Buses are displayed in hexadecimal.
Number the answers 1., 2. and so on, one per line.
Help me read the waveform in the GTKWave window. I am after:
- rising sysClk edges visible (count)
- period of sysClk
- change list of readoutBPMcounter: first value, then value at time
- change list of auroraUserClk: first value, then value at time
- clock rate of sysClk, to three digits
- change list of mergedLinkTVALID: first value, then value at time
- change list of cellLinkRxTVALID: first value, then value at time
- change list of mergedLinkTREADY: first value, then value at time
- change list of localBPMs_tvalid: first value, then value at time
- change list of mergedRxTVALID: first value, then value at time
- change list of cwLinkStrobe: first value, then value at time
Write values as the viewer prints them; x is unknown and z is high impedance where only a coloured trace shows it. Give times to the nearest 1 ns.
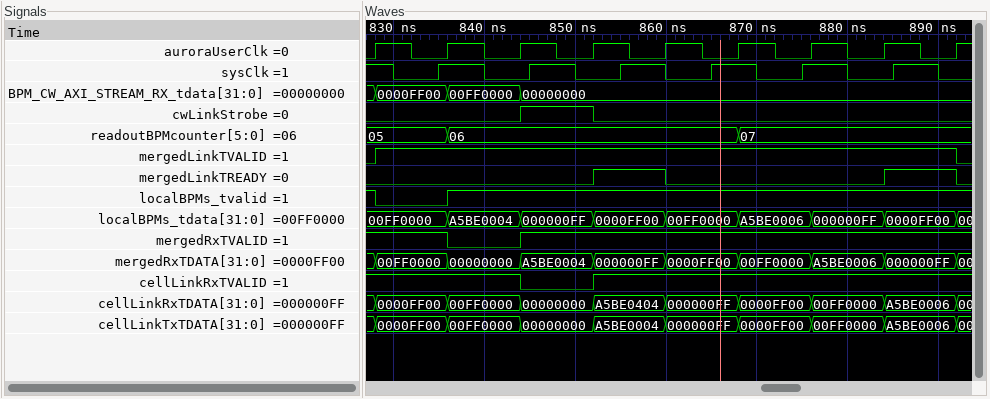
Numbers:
1. 6
2. 10 ns
3. 05, 06 at 836 ns, 07 at 868 ns
4. 0, 1 at 828 ns, 0 at 832 ns, 1 at 836 ns, 0 at 840 ns, 1 at 844 ns, 0 at 848 ns, 1 at 852 ns, 0 at 856 ns, 1 at 860 ns, 0 at 864 ns, 1 at 868 ns, 0 at 872 ns, 1 at 876 ns, 0 at 880 ns, 1 at 884 ns, 0 at 888 ns, 1 at 892 ns
5. 100 MHz
6. 0, 1 at 828 ns, 0 at 892 ns
7. 1, 0 at 844 ns, 1 at 852 ns
8. 0, 1 at 852 ns, 0 at 860 ns, 1 at 884 ns, 0 at 892 ns
9. 1, 0 at 828 ns, 1 at 836 ns
10. 1, 0 at 836 ns, 1 at 844 ns
11. 0, 1 at 844 ns, 0 at 852 ns
